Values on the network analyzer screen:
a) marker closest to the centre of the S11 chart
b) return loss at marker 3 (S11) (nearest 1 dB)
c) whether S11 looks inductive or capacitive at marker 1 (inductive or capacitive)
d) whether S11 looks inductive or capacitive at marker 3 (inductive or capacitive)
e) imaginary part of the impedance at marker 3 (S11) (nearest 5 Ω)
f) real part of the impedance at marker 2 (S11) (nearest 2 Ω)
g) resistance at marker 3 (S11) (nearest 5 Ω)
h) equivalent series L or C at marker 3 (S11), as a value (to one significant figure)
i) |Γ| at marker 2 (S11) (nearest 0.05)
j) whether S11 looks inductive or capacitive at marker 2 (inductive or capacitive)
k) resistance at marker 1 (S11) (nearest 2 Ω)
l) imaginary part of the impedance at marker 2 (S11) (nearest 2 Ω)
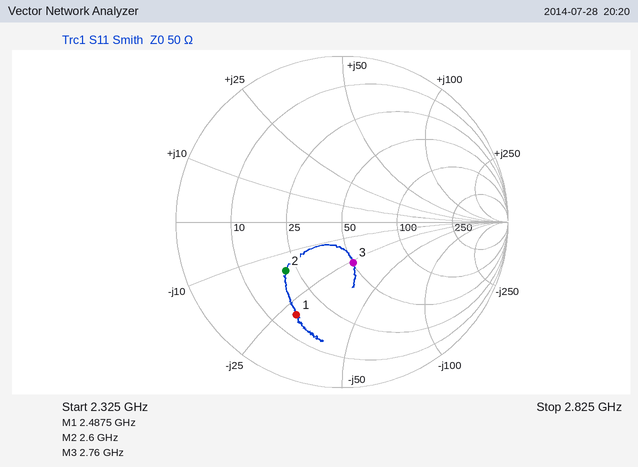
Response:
marker 3
12 dB
capacitive
capacitive
-25 Ω
22 Ω
50 Ω
2 pF
0.45
capacitive
16 Ω
-16 Ω
